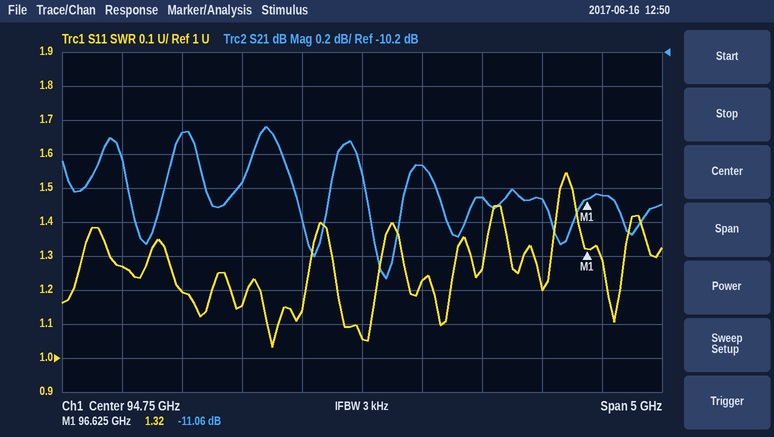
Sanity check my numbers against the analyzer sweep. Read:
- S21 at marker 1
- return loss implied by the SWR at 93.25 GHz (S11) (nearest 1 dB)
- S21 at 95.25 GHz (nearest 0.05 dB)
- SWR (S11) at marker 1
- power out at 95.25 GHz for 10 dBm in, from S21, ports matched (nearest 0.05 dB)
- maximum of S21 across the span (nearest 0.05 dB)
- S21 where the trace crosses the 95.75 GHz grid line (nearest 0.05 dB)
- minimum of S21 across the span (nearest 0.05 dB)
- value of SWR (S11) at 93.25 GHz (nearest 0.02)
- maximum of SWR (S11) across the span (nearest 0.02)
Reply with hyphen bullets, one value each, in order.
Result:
- -11.06 dB
- 21 dB
- -10.85 dB
- 1.32
- -0.85 dBm
- -10.65 dB
- -11.05 dB
- -11.55 dB
- 1.20
- 1.54
